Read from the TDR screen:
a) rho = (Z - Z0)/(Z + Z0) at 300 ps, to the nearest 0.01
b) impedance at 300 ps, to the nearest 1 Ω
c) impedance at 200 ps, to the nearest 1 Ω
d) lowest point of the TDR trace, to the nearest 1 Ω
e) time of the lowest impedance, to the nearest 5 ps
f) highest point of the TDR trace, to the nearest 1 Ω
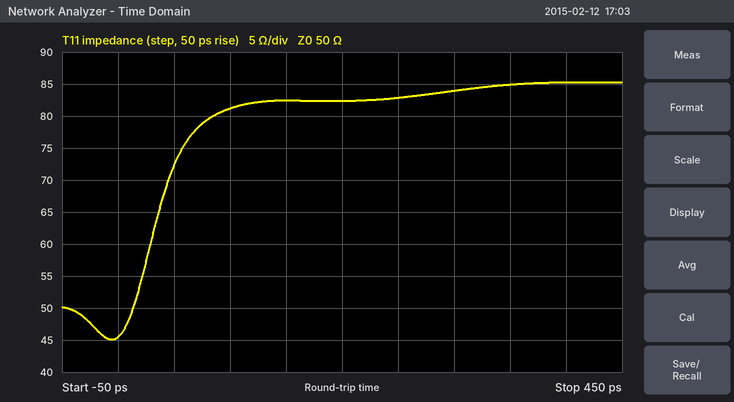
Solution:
+0.25
84 Ω
82 Ω
45 Ω
-5 ps
85 Ω
